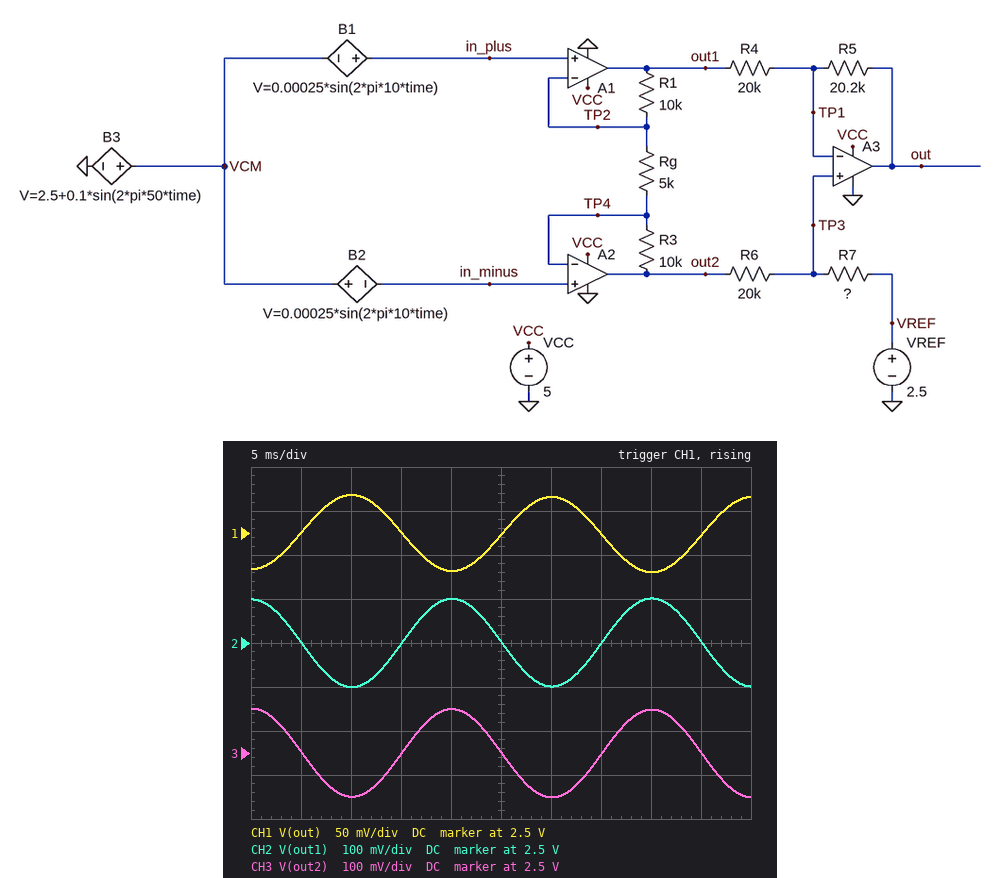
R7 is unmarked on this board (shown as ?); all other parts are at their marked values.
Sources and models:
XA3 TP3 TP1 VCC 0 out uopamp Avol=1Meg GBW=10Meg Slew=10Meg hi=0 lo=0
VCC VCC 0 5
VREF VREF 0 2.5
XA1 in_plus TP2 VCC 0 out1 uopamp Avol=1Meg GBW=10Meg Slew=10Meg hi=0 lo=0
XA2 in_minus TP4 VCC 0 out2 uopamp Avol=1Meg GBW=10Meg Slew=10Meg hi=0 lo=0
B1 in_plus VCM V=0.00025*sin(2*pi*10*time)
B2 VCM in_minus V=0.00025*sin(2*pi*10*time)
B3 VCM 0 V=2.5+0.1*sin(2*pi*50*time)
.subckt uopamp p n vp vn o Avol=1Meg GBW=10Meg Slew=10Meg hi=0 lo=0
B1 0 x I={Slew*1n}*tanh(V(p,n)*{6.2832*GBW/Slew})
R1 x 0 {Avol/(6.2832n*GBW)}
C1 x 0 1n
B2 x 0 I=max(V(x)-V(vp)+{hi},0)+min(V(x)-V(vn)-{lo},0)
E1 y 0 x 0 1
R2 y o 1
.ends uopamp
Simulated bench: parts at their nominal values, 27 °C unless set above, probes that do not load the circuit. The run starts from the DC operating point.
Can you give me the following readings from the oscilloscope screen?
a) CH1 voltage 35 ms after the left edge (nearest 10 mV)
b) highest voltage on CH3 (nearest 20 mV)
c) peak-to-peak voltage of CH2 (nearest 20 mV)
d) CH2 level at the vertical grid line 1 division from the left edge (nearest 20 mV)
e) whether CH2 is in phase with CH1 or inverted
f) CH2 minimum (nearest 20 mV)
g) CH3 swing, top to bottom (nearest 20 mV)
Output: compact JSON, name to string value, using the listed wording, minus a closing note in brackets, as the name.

{"CH1 voltage 35 ms after the left edge": "2.50 V", "highest voltage on CH3": "2.60 V", "peak-to-peak voltage of CH2": "200 mV", "CH2 level at the vertical grid line 1 division from the left edge": "2.50 V", "whether CH2 is in phase with CH1 or inverted": "inverted", "CH2 minimum": "2.40 V", "CH3 swing, top to bottom": "200 mV"}
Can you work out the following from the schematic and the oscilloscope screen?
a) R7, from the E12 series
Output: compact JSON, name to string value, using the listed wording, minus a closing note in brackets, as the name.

{"R7, from the E12 series": "8.2 kΩ"}
